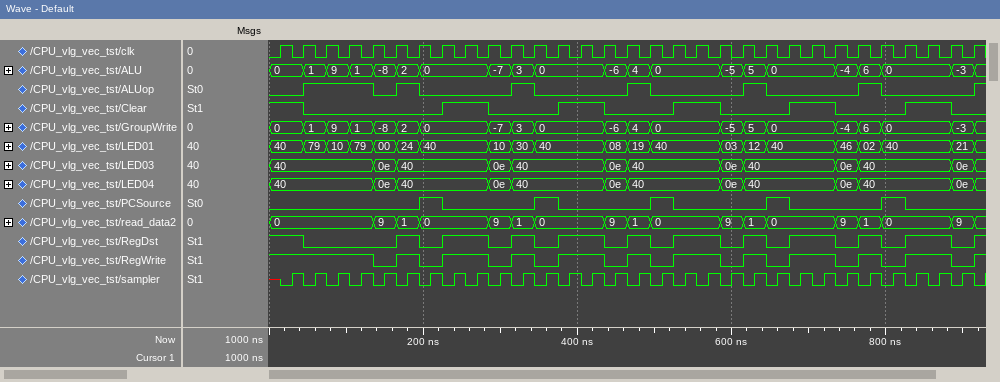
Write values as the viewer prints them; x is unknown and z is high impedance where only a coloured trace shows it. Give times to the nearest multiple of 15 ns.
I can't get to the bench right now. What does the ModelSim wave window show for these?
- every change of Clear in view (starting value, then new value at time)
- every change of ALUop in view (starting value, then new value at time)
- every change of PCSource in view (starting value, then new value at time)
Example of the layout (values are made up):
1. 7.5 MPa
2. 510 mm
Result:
1. 1, 0 at 45 ns, 1 at 225 ns, 0 at 285 ns, 1 at 375 ns, 0 at 435 ns, 1 at 525 ns, 0 at 585 ns, 1 at 675 ns, 0 at 735 ns, 1 at 825 ns, 0 at 885 ns
2. 0, 1 at 45 ns, 0 at 135 ns, 1 at 165 ns, 0 at 195 ns, 1 at 315 ns, 0 at 345 ns, 1 at 465 ns, 0 at 495 ns, 1 at 615 ns, 0 at 645 ns, 1 at 765 ns, 0 at 795 ns, 1 at 915 ns
3. 0, 1 at 195 ns, 0 at 225 ns, 1 at 345 ns, 0 at 375 ns, 1 at 495 ns, 0 at 525 ns, 1 at 645 ns, 0 at 675 ns, 1 at 795 ns, 0 at 825 ns
